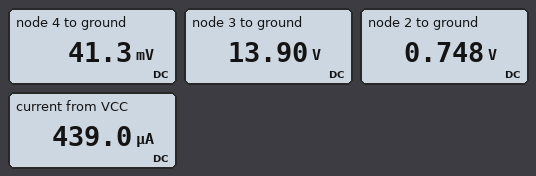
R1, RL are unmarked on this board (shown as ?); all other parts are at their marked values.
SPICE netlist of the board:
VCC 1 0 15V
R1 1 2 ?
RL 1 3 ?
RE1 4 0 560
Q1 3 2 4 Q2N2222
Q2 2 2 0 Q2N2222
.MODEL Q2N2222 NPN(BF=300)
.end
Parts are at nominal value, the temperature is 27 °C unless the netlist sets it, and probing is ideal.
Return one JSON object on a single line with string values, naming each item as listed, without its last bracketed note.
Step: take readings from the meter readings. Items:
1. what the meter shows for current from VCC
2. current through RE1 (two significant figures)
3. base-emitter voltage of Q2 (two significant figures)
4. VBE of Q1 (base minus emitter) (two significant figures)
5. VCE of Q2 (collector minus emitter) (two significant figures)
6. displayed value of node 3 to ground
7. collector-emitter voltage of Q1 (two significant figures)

{"what the meter shows for current from VCC": "439.0 µA", "current through RE1": "74 µA", "base-emitter voltage of Q2": "750 mV", "VBE of Q1 (base minus emitter)": "710 mV", "VCE of Q2 (collector minus emitter)": "750 mV", "displayed value of node 3 to ground": "13.90 V", "collector-emitter voltage of Q1": "14 V"}
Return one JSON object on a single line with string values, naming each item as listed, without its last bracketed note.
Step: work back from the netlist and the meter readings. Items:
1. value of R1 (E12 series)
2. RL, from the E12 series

{"value of R1": "39 kΩ", "RL, from the E12 series": "15 kΩ"}
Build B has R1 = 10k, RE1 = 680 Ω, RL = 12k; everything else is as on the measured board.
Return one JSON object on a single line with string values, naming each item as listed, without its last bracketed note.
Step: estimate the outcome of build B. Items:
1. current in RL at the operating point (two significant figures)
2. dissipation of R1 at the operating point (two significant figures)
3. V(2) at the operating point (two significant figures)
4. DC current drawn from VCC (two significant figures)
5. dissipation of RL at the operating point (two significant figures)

{"current in RL at the operating point": "100 µA", "dissipation of R1 at the operating point": "20 mW", "V(2) at the operating point": "780 mV", "DC current drawn from VCC": "1.5 mA", "dissipation of RL at the operating point": "120 µW"}
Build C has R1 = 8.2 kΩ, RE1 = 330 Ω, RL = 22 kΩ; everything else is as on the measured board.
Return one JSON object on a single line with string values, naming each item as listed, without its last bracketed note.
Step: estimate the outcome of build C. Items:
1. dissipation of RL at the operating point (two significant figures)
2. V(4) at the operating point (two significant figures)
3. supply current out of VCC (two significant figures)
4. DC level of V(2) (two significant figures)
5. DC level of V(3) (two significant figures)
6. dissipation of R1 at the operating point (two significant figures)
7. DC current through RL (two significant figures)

{"dissipation of RL at the operating point": "690 µW", "V(4) at the operating point": "59 mV", "supply current out of VCC": "1.9 mA", "DC level of V(2)": "790 mV", "DC level of V(3)": "11 V", "dissipation of R1 at the operating point": "25 mW", "DC current through RL": "180 µA"}
